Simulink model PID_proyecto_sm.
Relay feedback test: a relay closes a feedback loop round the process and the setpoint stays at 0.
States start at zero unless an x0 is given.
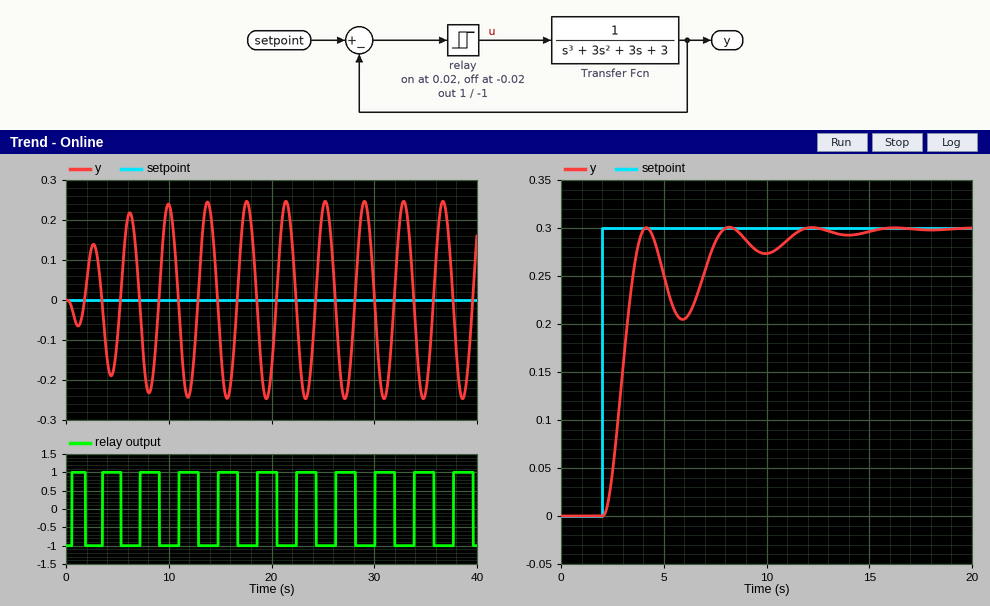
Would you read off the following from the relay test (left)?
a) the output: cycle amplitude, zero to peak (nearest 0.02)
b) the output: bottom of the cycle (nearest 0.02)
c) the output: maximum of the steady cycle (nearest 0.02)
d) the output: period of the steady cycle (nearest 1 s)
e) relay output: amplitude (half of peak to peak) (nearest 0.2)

0.24
-0.24
0.24
4 s
1.0
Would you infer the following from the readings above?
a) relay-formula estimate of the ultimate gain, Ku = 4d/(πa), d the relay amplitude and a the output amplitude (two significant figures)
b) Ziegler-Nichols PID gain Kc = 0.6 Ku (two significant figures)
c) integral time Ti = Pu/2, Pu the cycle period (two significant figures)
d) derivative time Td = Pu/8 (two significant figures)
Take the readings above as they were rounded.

5.3
3.2
2.0 s
0.50 s
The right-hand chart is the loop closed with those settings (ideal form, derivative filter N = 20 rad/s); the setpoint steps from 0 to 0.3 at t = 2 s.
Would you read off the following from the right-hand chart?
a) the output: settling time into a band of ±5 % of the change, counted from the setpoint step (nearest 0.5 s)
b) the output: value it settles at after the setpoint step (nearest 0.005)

9.0 s
0.300
